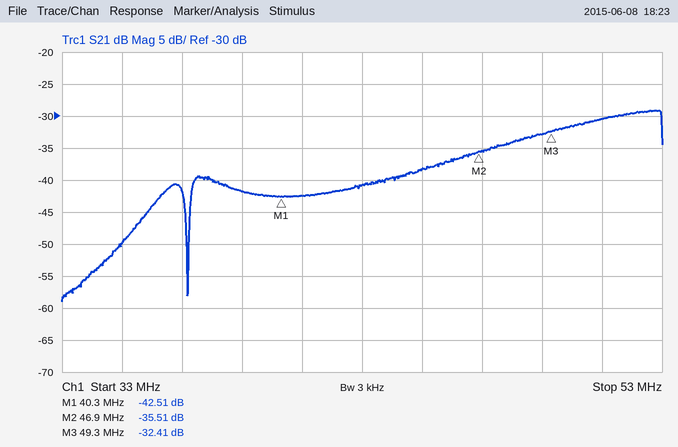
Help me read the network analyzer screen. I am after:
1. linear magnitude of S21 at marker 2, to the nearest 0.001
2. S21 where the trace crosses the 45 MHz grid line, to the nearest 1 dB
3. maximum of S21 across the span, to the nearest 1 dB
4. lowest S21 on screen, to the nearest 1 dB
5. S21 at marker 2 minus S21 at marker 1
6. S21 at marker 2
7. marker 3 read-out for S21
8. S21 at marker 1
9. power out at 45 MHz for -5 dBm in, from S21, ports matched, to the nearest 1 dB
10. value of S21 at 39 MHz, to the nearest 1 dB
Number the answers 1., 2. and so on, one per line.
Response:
1. 0.017
2. -38 dB
3. -29 dB
4. -59 dB
5. 7.00 dB
6. -35.51 dB
7. -32.41 dB
8. -42.51 dB
9. -43 dBm
10. -42 dB
